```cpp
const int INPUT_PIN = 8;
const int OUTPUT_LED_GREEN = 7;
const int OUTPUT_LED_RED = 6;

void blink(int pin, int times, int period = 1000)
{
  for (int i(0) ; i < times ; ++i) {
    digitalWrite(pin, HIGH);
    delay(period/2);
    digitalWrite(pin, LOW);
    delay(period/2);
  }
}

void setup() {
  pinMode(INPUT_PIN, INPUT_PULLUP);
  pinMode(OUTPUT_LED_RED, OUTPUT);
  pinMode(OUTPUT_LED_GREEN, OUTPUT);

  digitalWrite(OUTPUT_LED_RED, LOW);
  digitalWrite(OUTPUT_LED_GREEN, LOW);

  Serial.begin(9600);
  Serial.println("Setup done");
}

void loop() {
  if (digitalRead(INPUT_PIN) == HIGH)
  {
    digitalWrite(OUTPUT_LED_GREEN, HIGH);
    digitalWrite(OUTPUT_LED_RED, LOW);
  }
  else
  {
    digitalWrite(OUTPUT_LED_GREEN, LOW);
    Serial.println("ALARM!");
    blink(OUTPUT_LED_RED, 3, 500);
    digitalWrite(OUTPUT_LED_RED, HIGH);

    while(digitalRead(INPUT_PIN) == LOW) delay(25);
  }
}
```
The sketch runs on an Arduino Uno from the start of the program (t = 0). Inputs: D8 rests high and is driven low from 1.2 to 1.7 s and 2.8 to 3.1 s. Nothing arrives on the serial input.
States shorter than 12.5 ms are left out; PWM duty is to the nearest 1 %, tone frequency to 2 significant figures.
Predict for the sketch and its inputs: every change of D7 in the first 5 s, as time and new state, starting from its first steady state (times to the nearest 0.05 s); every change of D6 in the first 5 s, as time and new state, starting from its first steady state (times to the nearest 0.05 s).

0 s high; 1.2 s low; 2.7 s high; 2.8 s low; 4.3 s high
0 s low; 1.2 s high; 1.45 s low; 1.7 s high; 1.95 s low; 2.2 s high; 2.45 s low; 2.8 s high; 3.05 s low; 3.3 s high; 3.55 s low; 3.8 s high; 4.05 s low
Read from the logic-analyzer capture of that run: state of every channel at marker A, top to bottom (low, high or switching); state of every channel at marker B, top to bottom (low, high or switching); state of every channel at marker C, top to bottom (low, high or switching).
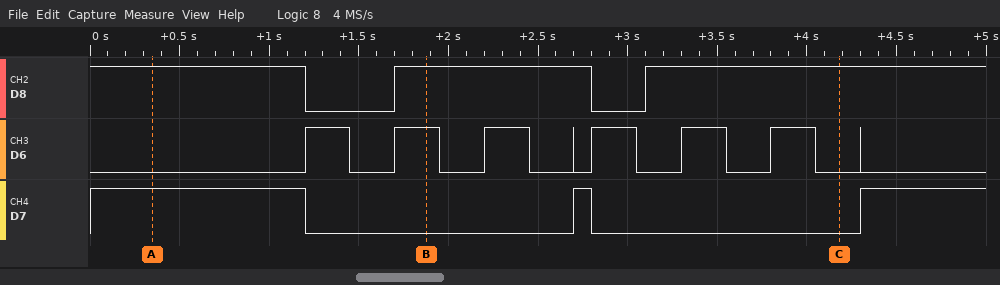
D8 high, D6 low, D7 high
D8 high, D6 high, D7 low
D8 high, D6 low, D7 low
